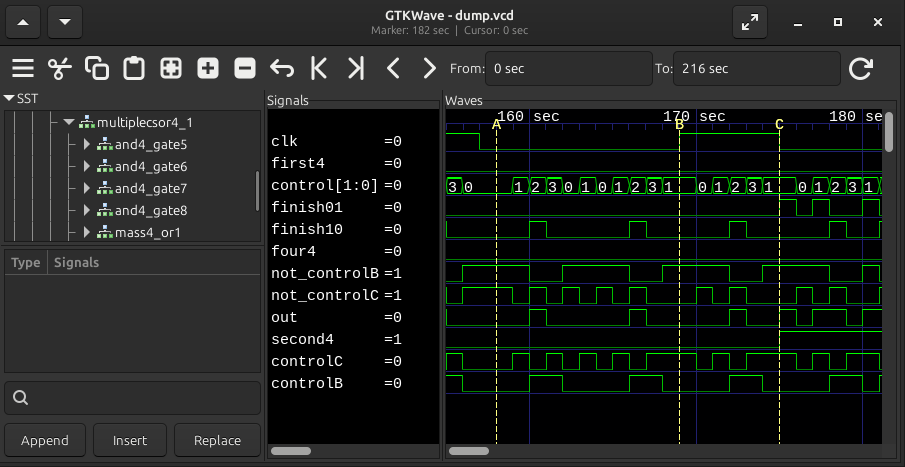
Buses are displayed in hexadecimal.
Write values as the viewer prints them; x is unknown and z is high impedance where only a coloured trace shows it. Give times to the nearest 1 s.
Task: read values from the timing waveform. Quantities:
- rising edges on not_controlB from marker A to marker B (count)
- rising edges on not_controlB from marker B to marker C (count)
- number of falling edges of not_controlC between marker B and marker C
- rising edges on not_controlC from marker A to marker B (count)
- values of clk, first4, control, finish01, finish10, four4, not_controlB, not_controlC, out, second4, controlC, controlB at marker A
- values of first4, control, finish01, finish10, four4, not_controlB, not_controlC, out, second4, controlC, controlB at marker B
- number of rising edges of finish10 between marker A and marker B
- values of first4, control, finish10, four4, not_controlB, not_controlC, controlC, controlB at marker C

2
1
2
4
clk=0, first4=0, control=0, finish01=0, finish10=0, four4=0, not_controlB=1, not_controlC=1, out=0, second4=0, controlC=0, controlB=0
first4=0, control=1, finish01=0, finish10=0, four4=0, not_controlB=1, not_controlC=0, out=0, second4=0, controlC=1, controlB=0
2
first4=0, control=1, finish10=0, four4=0, not_controlB=1, not_controlC=0, controlC=1, controlB=0
